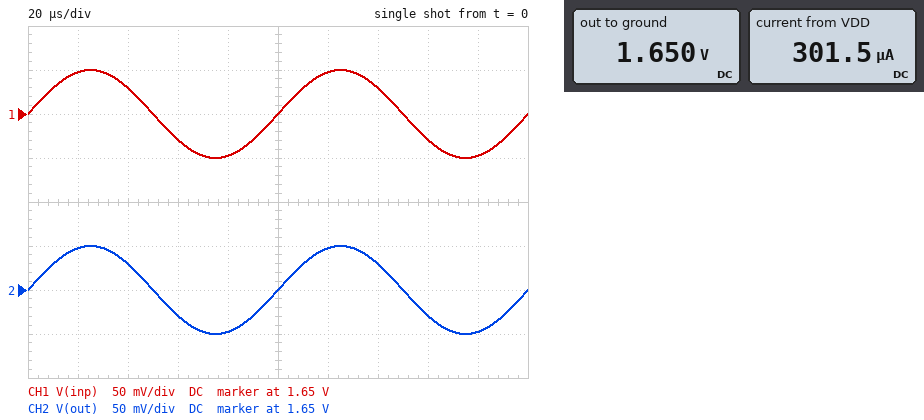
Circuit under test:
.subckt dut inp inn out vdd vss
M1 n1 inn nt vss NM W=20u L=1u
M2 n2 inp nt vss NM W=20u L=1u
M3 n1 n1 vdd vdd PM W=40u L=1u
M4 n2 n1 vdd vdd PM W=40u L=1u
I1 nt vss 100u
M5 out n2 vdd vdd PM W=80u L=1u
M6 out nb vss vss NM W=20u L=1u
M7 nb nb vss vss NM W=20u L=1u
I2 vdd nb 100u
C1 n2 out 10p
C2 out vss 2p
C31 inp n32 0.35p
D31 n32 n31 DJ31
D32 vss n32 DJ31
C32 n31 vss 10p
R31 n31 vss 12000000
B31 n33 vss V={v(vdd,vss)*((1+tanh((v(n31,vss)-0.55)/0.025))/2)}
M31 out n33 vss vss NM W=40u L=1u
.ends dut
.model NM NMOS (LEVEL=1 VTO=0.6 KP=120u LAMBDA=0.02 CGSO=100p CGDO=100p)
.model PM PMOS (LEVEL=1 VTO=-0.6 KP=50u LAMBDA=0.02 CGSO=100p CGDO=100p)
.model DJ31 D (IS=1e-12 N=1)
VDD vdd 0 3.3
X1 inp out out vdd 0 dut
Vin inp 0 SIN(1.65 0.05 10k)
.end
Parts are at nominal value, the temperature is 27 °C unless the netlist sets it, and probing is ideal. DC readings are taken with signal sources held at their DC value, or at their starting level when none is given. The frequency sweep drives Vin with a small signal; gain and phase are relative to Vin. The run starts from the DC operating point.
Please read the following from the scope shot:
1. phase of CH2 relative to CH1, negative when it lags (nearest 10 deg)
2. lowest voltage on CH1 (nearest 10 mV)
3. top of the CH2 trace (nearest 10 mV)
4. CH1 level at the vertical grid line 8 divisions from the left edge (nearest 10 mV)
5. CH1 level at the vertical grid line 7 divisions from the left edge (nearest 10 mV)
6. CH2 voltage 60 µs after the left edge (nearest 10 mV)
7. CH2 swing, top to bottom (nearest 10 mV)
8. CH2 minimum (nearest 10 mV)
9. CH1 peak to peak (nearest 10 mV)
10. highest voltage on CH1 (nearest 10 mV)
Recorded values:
0 deg
1.60 V
1.70 V
1.62 V
1.68 V
1.62 V
100 mV
1.60 V
100 mV
1.70 V
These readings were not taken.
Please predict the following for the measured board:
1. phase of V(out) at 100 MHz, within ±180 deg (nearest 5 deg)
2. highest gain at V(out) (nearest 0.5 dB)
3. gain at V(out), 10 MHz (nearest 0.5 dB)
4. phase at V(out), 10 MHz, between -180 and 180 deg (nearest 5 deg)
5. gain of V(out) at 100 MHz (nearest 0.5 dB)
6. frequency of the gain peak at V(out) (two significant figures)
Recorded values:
115 deg
3.0 dB
1.5 dB
-70 deg
-8.0 dB
20 MHz
